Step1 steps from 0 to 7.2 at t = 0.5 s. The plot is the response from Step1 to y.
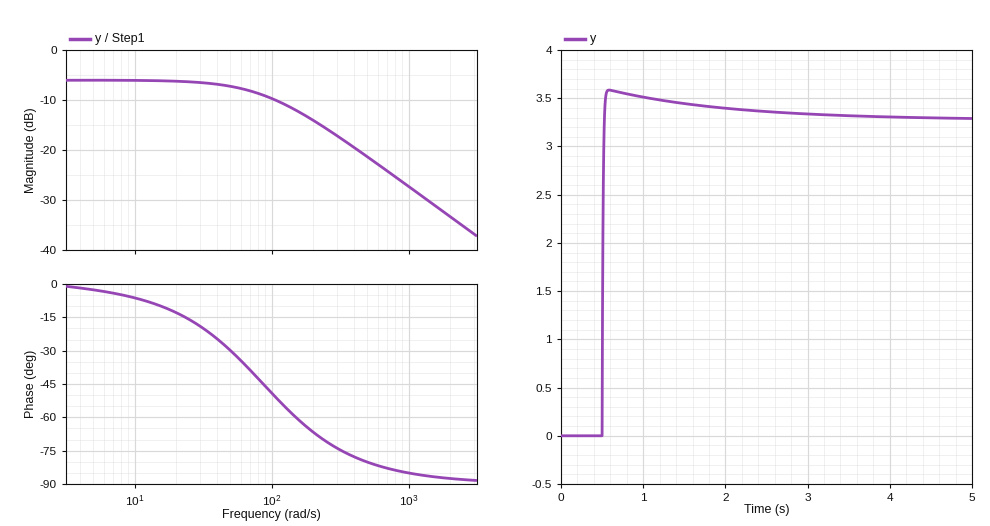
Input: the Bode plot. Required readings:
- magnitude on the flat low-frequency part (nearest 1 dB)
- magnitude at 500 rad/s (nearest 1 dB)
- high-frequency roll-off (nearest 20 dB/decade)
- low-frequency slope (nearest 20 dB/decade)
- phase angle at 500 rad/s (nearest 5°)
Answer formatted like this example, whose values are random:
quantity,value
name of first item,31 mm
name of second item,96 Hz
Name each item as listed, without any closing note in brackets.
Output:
quantity,value
magnitude on the flat low-frequency part,-6 dB
magnitude at 500 rad/s,-21 dB
high-frequency roll-off,-20 dB/decade
low-frequency slope,0 dB/decade
phase angle at 500 rad/s,-80°
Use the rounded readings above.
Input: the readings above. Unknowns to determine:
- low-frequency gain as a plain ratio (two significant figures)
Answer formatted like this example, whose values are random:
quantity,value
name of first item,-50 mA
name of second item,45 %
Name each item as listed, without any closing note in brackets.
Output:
quantity,value
low-frequency gain as a plain ratio,0.50
